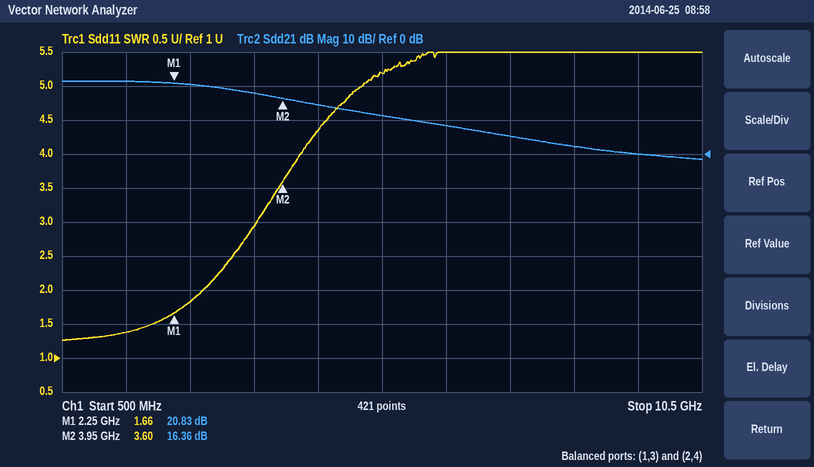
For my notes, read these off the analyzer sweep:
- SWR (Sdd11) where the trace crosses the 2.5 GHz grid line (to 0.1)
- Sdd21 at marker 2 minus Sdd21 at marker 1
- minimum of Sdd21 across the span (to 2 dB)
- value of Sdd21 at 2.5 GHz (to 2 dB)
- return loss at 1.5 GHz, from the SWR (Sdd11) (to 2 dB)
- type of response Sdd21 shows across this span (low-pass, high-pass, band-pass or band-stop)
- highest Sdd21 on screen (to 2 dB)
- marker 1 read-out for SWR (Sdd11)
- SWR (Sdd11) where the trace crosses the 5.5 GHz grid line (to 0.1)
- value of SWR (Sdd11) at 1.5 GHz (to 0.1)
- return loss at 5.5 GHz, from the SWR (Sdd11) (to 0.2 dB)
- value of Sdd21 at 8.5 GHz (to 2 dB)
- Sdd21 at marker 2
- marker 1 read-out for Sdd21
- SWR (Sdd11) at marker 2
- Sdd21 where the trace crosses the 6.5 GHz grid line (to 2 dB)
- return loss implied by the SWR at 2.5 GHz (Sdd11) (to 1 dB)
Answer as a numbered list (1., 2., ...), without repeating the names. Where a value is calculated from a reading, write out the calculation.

1. 1.8
2. 16.36 − (20.83) = -4.47 dB
3. -2 dB
4. 20 dB
5. −20 log10((1.4 − 1)/(1.4 + 1)) ≈ 16 dB
6. low-pass
7. 22 dB
8. 1.66
9. 5.2
10. 1.4
11. −20 log10((5.2 − 1)/(5.2 + 1)) ≈ 3.4 dB
12. 2 dB
13. 16.36 dB
14. 20.83 dB
15. 3.60
16. 8 dB
17. −20 log10((1.8 − 1)/(1.8 + 1)) ≈ 11 dB
